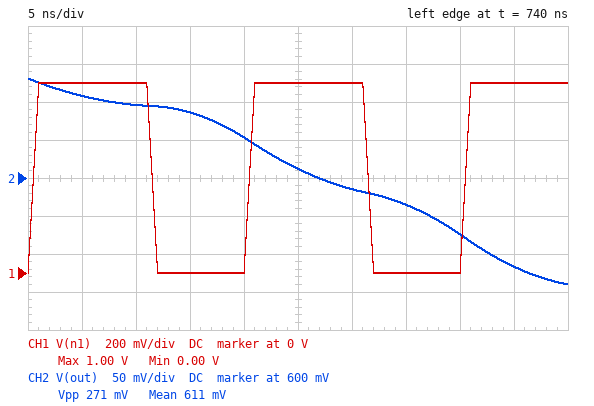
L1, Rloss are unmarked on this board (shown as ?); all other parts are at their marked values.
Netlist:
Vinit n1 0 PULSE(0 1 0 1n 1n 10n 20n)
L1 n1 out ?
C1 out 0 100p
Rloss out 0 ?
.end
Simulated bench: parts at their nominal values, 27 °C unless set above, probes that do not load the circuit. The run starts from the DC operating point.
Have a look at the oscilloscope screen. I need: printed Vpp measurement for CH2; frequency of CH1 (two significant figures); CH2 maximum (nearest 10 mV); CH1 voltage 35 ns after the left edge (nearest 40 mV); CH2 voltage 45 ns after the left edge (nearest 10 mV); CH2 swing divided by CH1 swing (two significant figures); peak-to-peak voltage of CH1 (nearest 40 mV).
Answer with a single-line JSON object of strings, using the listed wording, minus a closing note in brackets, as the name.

{"printed Vpp measurement for CH2": "271 mV", "frequency of CH1": "50 MHz", "CH2 maximum": "730 mV", "CH1 voltage 35 ns after the left edge": "0 V", "CH2 voltage 45 ns after the left edge": "480 mV", "CH2 swing divided by CH1 swing": "0.27", "peak-to-peak voltage of CH1": "1.00 V"}
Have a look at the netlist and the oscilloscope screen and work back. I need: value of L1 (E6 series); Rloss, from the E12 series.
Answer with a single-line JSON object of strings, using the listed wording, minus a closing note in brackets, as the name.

{"value of L1": "6.8 µH", "Rloss, from the E12 series": "3.3 kΩ"}
